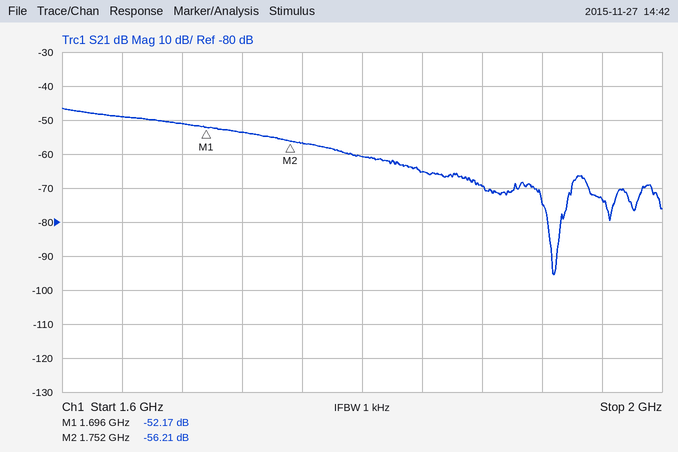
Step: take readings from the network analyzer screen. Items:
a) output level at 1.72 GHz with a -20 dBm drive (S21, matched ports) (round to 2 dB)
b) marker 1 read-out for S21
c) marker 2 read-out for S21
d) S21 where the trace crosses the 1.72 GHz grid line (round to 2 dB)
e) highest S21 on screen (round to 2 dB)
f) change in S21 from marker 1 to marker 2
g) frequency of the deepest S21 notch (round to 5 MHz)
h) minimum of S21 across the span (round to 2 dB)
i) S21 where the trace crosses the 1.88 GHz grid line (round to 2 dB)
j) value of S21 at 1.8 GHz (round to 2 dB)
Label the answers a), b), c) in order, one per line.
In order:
a) -74 dBm
b) -52.17 dB
c) -56.21 dB
d) -54 dB
e) -46 dB
f) -4.04 dB
g) 1.930 GHz
h) -96 dB
i) -70 dB
j) -60 dB
